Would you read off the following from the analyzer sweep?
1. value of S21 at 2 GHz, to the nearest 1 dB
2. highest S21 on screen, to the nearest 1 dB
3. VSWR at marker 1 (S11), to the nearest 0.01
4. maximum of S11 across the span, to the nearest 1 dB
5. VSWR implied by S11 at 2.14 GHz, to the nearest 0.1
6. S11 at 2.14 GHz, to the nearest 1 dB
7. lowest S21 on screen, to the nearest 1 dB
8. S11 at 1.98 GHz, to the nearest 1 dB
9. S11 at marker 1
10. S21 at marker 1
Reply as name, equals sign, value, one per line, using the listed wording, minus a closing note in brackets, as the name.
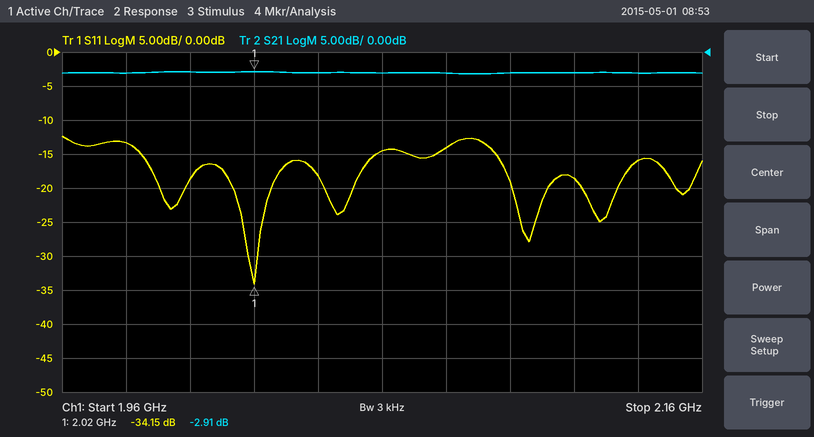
value of S21 at 2 GHz, to the nearest 1 dB = -3 dB
highest S21 on screen, to the nearest 1 dB = -3 dB
VSWR at marker 1 (S11), to the nearest 0.01 = 1.04
maximum of S11 across the span, to the nearest 1 dB = -12 dB
VSWR implied by S11 at 2.14 GHz, to the nearest 0.1 = 1.4
S11 at 2.14 GHz, to the nearest 1 dB = -16 dB
lowest S21 on screen, to the nearest 1 dB = -3 dB
S11 at 1.98 GHz, to the nearest 1 dB = -13 dB
S11 at marker 1 = -34.15 dB
S21 at marker 1 = -2.91 dB
